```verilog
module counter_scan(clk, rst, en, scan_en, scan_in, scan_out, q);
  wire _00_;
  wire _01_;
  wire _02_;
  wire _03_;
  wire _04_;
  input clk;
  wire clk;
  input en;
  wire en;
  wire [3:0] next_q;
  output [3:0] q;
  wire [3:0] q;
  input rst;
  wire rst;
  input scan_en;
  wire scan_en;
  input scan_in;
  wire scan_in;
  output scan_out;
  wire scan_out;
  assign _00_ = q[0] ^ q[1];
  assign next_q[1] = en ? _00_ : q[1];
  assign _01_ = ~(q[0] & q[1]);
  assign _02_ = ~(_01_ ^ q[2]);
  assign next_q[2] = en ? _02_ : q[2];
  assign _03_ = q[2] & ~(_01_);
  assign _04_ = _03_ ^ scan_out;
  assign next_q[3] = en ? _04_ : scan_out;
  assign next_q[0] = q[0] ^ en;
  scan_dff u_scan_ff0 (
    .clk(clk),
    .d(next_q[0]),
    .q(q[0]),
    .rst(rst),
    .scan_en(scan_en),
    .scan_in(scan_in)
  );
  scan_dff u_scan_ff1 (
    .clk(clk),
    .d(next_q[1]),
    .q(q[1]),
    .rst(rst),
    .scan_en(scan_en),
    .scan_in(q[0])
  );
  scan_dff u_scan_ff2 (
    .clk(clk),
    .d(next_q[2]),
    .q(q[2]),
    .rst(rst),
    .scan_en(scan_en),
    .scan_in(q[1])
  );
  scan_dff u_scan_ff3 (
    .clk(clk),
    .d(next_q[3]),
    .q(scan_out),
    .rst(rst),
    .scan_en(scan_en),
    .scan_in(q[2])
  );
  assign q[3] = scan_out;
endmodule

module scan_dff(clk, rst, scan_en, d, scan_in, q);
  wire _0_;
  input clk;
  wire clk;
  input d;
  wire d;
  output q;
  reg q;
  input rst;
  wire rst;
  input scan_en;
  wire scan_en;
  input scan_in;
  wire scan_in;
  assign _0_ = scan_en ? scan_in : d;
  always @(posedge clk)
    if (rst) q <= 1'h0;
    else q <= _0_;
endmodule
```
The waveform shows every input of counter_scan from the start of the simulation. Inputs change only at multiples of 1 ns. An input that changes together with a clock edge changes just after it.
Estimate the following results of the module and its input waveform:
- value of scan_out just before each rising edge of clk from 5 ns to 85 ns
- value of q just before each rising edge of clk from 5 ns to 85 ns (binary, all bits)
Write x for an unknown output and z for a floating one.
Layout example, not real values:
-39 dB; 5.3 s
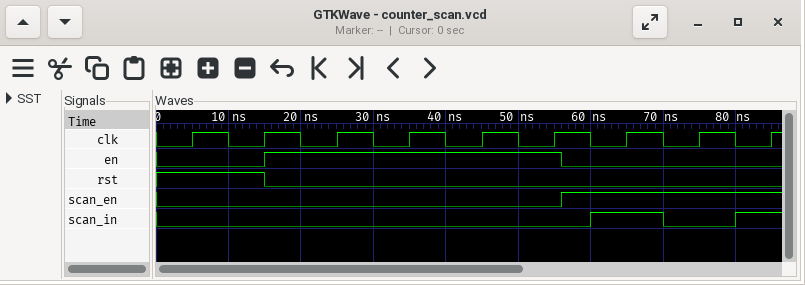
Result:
x 0 0 0 0 0 0 1 0; x, 0000, 0000, 0001, 0010, 0011, 0100, 1001, 0010
